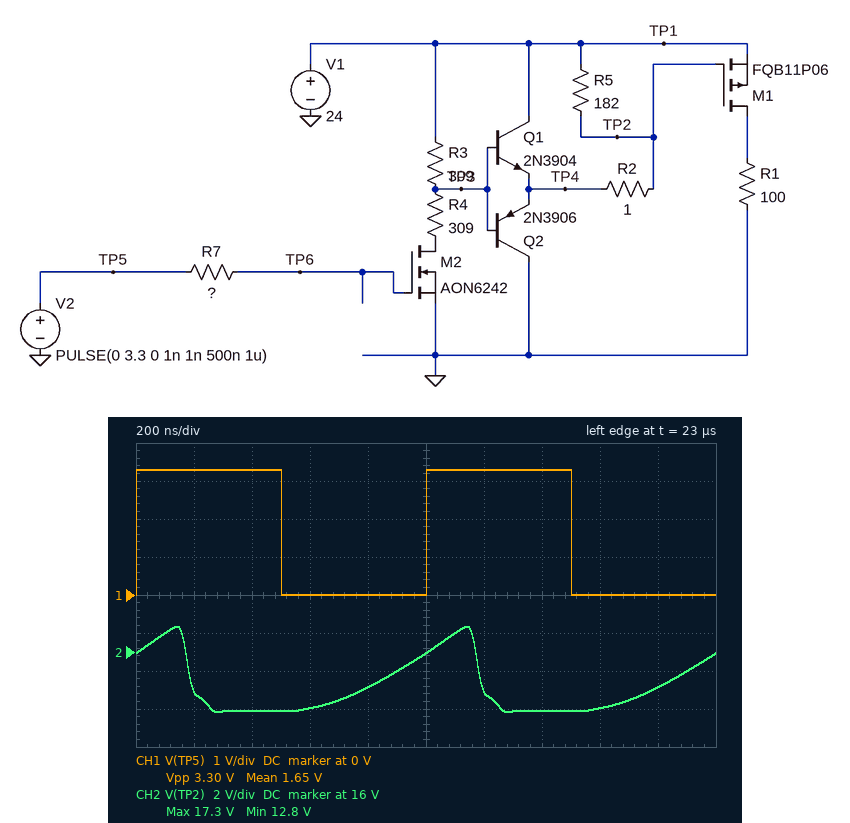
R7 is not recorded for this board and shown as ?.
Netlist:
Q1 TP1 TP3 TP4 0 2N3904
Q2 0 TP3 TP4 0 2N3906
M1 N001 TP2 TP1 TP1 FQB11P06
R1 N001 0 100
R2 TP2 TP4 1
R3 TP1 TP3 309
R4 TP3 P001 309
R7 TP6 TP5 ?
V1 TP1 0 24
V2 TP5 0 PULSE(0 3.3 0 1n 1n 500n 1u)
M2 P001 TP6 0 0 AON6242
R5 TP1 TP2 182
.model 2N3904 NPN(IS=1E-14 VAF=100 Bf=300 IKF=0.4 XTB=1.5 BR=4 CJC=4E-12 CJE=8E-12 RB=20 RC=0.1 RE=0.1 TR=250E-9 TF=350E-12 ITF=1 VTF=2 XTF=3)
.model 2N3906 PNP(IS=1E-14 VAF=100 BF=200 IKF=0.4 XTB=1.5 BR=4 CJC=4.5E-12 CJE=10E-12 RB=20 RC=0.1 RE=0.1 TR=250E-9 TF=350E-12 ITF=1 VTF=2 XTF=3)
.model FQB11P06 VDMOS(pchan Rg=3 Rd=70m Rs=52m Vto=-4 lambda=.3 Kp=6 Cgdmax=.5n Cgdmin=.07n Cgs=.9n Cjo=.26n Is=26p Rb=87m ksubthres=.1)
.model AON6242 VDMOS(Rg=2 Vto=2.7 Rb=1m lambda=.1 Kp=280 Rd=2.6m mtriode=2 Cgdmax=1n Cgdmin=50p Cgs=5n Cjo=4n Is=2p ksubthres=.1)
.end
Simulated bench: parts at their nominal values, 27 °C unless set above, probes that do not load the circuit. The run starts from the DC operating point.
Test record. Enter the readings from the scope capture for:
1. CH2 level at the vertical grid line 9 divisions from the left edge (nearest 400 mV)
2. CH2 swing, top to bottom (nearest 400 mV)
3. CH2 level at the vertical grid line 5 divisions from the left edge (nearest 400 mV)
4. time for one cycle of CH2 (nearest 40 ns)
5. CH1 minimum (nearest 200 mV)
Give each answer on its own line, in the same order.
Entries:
14.0 V
4.4 V
16.0 V
1.00 µs
0 V
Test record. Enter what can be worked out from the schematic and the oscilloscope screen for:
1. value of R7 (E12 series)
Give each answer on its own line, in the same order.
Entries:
18 Ω
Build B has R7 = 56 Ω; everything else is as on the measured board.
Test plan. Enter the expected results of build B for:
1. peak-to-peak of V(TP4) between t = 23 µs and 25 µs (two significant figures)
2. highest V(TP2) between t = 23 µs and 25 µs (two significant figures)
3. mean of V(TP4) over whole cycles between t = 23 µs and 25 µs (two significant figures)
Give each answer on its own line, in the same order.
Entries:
6.6 V
21 V
18 V
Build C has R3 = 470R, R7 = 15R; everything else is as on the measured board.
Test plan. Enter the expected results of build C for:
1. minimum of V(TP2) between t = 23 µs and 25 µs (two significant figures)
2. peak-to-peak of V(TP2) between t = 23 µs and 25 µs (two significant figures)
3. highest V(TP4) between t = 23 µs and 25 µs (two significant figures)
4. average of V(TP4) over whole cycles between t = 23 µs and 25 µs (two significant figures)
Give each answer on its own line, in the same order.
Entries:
10 V
3.9 V
14 V
11 V
